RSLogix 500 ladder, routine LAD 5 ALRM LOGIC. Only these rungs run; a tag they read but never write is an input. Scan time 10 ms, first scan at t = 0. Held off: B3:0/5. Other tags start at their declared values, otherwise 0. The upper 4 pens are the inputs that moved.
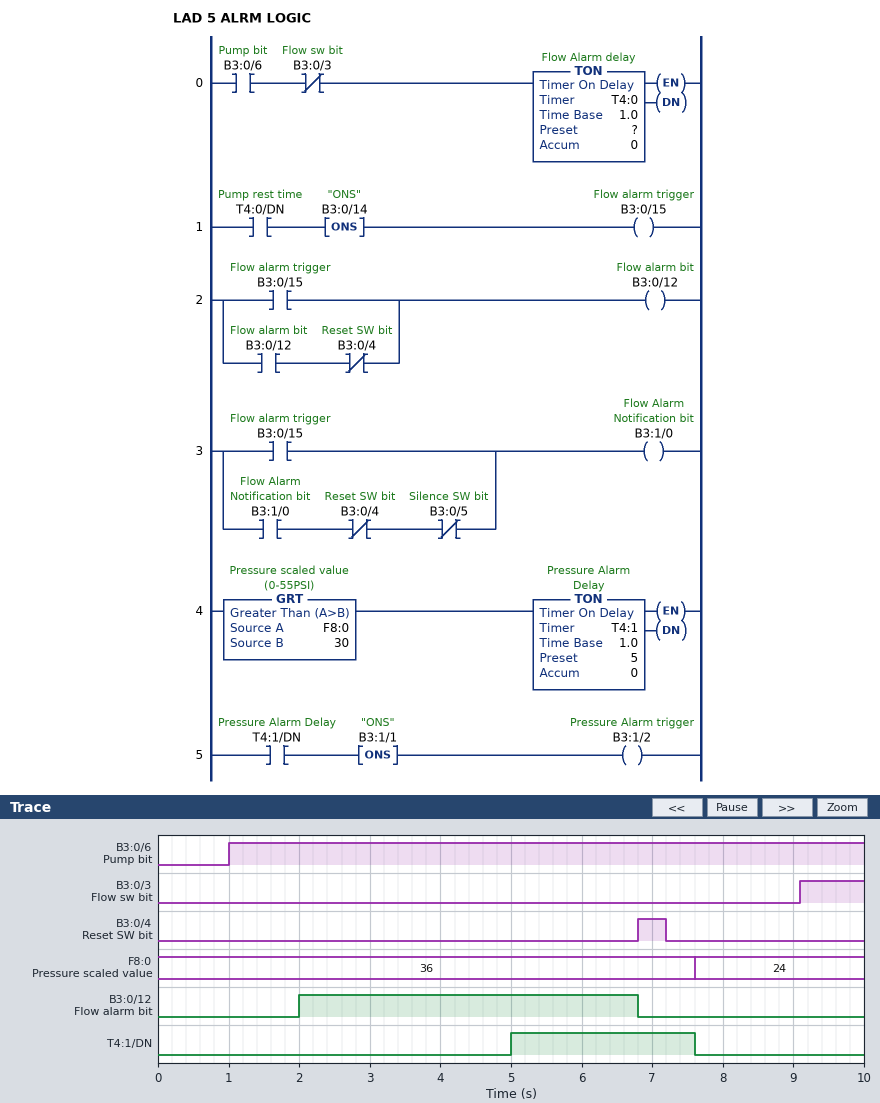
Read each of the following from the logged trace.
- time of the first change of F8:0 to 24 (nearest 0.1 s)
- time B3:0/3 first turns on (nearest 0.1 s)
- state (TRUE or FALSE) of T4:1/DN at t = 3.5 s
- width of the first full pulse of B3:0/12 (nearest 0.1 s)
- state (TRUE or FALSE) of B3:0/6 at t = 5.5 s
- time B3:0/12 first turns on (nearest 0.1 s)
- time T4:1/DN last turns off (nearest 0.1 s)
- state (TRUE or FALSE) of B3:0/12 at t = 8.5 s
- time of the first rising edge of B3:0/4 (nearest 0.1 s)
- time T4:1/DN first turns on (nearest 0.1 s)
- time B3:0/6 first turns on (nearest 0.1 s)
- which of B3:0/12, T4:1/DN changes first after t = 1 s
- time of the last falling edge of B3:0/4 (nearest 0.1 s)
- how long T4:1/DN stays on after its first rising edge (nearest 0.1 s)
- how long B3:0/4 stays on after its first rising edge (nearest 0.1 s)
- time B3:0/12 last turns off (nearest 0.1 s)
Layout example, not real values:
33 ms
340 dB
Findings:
7.6 s
9.1 s
FALSE
4.8 s
TRUE
2.0 s
7.6 s
FALSE
6.8 s
5.0 s
1.0 s
B3:0/12
7.2 s
2.6 s
0.4 s
6.8 s
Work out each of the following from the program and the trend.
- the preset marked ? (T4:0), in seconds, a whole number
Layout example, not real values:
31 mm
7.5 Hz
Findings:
1 s
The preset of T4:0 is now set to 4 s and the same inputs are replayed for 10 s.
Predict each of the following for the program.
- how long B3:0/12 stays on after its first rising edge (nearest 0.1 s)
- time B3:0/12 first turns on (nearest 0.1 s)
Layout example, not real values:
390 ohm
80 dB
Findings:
1.8 s
5.0 s
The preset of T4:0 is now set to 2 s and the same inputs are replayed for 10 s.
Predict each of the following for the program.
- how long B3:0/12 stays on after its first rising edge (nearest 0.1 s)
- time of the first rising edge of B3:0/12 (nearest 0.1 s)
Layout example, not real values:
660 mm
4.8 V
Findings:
3.8 s
3.0 s
